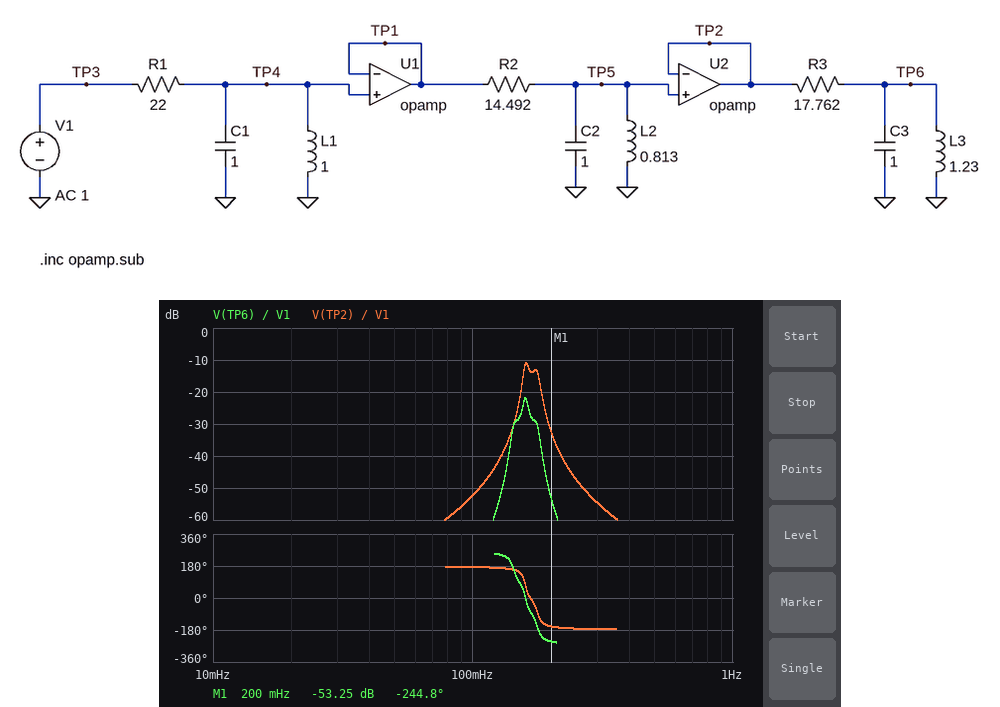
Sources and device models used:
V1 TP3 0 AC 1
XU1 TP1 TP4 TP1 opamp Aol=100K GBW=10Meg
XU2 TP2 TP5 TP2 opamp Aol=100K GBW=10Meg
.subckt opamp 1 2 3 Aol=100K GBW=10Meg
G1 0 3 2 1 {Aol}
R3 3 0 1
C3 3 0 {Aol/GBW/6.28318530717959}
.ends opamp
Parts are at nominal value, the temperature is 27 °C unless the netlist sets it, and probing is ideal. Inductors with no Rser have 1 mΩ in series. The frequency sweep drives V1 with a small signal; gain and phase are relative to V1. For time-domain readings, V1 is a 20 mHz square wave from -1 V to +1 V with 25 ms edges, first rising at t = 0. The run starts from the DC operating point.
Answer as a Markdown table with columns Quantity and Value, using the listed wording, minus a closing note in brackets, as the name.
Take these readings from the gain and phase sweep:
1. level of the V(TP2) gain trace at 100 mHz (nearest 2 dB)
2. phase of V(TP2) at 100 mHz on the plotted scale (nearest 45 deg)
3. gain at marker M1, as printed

| Quantity | Value |
|---|---|
| level of the V(TP2) gain trace at 100 mHz | -52 dB |
| phase of V(TP2) at 100 mHz on the plotted scale | 180 deg |
| gain at marker M1, as printed | -53.25 dB |
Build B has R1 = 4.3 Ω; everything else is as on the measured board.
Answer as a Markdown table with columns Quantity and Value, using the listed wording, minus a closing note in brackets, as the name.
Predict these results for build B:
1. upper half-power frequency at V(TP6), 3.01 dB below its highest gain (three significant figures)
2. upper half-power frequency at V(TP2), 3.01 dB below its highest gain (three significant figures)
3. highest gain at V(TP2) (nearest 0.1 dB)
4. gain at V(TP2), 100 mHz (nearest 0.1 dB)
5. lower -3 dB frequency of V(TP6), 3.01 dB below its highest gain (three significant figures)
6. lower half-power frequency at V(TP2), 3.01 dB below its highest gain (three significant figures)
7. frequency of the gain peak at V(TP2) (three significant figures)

| Quantity | Value |
|---|---|
| upper half-power frequency at V(TP6), 3.01 dB below its highest gain | 180 mHz |
| upper half-power frequency at V(TP2), 3.01 dB below its highest gain | 181 mHz |
| highest gain at V(TP2) | -2.6 dB |
| gain at V(TP2), 100 mHz | -38.3 dB |
| lower -3 dB frequency of V(TP6), 3.01 dB below its highest gain | 141 mHz |
| lower half-power frequency at V(TP2), 3.01 dB below its highest gain | 169 mHz |
| frequency of the gain peak at V(TP2) | 176 mHz |
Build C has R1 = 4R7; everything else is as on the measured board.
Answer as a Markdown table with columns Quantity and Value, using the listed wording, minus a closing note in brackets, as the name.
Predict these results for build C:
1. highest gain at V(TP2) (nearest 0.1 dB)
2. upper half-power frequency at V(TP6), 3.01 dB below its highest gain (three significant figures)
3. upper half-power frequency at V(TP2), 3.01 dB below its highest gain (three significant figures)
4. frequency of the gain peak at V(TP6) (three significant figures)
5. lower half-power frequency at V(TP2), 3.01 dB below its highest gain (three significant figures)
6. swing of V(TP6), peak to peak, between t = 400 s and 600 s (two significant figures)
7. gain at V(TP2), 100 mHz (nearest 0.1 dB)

| Quantity | Value |
|---|---|
| highest gain at V(TP2) | -3.0 dB |
| upper half-power frequency at V(TP6), 3.01 dB below its highest gain | 180 mHz |
| upper half-power frequency at V(TP2), 3.01 dB below its highest gain | 181 mHz |
| frequency of the gain peak at V(TP6) | 175 mHz |
| lower half-power frequency at V(TP2), 3.01 dB below its highest gain | 169 mHz |
| swing of V(TP6), peak to peak, between t = 400 s and 600 s | 44 mV |
| gain at V(TP2), 100 mHz | -39.0 dB |
